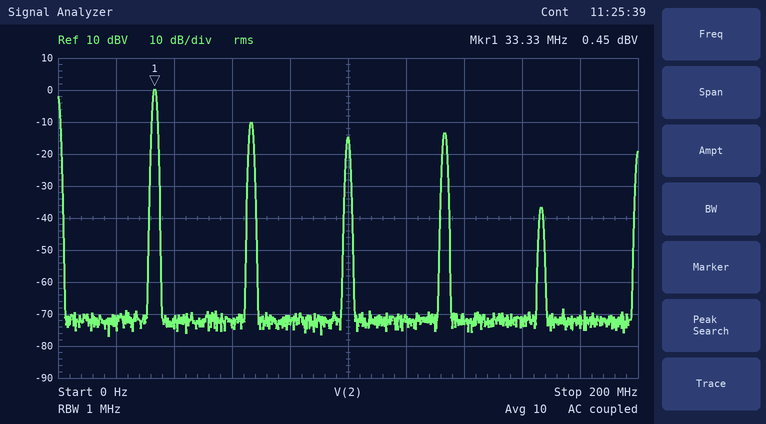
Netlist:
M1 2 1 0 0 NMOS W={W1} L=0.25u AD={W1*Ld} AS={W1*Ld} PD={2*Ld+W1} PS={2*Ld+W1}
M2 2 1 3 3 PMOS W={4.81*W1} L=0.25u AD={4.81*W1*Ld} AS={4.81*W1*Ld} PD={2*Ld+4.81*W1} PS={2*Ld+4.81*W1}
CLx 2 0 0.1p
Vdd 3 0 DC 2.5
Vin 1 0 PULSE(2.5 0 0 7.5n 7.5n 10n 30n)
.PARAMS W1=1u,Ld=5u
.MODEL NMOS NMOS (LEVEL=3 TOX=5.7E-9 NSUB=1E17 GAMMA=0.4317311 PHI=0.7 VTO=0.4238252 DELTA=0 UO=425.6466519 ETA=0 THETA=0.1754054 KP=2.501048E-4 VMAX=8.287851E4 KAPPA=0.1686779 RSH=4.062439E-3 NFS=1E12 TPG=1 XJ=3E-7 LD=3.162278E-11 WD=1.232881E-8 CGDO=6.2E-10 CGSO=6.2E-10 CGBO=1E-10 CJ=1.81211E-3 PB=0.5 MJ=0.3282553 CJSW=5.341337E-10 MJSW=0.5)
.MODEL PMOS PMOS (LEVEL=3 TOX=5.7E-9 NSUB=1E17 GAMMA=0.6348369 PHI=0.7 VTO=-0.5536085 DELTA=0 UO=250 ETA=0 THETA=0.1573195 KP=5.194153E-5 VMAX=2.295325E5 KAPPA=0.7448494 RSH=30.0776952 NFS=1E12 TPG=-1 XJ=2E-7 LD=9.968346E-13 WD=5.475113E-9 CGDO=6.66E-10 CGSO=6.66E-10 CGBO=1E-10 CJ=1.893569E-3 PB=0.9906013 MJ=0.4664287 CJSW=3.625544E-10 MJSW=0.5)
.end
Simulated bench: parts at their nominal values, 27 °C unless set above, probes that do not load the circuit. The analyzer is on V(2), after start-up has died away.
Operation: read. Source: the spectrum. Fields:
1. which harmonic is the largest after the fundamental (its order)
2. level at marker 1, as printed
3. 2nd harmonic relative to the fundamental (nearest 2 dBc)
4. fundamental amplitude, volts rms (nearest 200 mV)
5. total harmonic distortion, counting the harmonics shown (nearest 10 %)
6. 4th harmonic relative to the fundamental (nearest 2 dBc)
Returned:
2
0.45 dBV
-10 dBc
1.0 V
40 %
-14 dBc
